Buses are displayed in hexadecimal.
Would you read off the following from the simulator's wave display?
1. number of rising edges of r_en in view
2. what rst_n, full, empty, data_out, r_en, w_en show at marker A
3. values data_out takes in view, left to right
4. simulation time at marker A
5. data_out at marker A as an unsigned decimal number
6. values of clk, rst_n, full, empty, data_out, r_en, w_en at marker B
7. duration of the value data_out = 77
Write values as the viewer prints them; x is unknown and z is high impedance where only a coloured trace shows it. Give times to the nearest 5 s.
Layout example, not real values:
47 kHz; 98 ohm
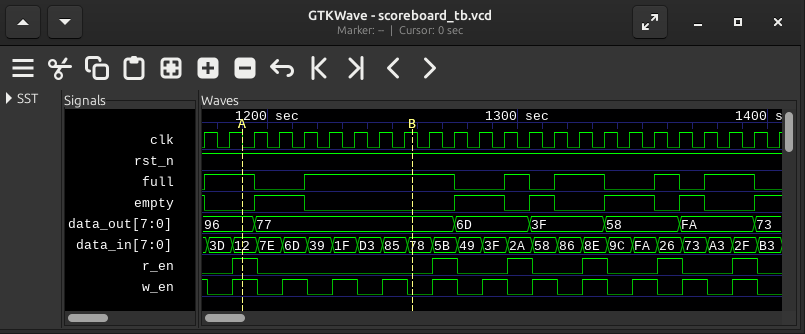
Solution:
6; rst_n=1, full=1, empty=0, data_out=96, r_en=1, w_en=1; 96, 77, 6D, 3F, 58, FA, 73; 1190 s; 150; clk=1, rst_n=1, full=1, empty=0, data_out=77, r_en=0, w_en=0; 80 s
